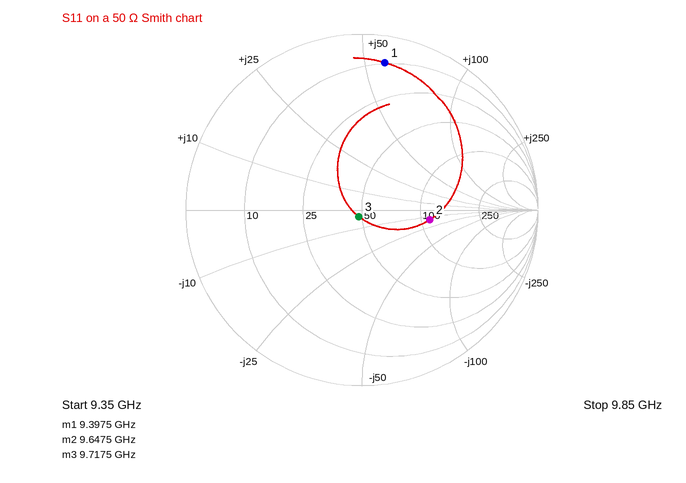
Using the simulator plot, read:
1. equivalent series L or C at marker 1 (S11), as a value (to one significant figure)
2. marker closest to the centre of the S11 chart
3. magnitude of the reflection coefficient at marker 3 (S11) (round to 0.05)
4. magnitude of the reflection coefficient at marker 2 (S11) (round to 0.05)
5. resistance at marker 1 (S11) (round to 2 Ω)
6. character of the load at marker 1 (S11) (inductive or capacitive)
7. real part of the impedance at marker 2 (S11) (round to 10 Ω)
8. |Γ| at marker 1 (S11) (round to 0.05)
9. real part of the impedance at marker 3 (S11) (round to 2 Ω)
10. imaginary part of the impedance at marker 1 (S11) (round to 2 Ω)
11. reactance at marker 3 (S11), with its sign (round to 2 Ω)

1.0 nH
marker 3
0.05
0.40
10 Ω
inductive
110 Ω
0.85
48 Ω
+58 Ω
-4 Ω
